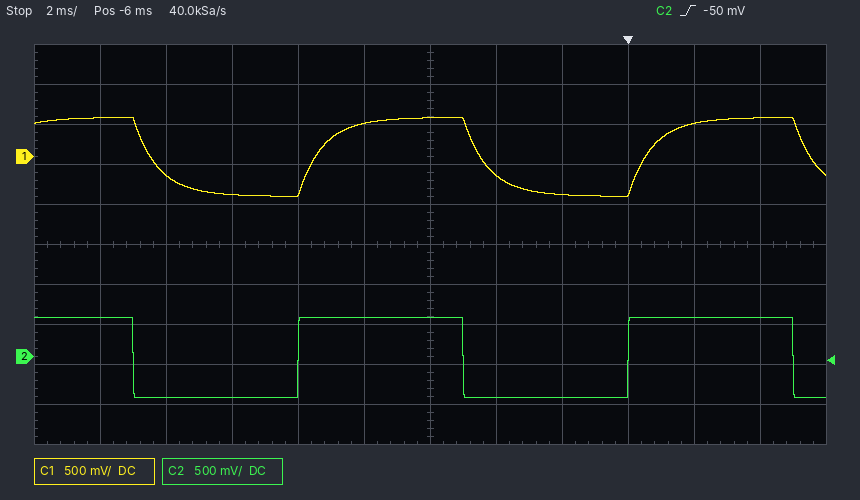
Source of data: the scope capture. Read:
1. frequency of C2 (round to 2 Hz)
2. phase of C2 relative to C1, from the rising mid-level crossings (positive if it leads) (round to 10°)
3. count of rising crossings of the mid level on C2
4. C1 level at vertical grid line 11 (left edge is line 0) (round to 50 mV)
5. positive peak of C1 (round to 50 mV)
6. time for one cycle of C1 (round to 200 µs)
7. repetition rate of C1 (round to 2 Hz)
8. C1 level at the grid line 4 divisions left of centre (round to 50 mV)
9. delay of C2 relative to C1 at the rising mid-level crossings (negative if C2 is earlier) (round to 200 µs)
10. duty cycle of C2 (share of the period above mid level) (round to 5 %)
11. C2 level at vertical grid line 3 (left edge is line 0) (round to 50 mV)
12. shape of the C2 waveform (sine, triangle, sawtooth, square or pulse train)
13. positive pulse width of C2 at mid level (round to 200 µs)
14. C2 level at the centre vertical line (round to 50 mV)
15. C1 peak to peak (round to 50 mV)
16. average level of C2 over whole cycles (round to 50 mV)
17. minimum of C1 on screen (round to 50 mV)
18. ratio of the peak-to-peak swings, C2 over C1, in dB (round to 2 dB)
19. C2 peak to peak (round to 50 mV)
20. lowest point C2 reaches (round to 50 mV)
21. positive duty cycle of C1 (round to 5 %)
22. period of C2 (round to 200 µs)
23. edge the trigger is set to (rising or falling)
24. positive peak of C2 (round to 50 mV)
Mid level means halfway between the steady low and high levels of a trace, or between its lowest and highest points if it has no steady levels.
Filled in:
100 Hz
+20°
2
500 mV
500 mV
10.0 ms
100 Hz
-250 mV
-600 µs
50 %
-500 mV
square
5.0 ms
500 mV
1.00 V
0 mV
-500 mV
0 dB
1.00 V
-500 mV
50 %
10.0 ms
rising
500 mV
